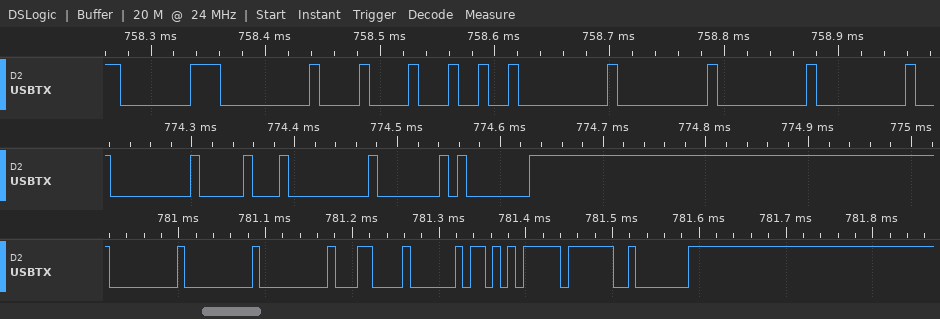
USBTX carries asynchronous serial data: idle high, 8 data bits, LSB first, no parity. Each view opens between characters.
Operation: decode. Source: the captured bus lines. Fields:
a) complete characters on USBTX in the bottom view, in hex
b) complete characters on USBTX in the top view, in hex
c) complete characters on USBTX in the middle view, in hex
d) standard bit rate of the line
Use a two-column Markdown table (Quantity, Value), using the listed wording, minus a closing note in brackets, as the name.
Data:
| Quantity | Value |
|---|---|
| complete characters on USBTX in the bottom view, in hex | 00, 00, 00, 0C, A0, F5, 3F, C0 |
| complete characters on USBTX in the top view, in hex | C0, 00, 08, 24, 00, 00, 00, 00 |
| complete characters on USBTX in the middle view, in hex | 00, 10, 00, 40, C0 |
| standard bit rate of the line | 115200 baud |
